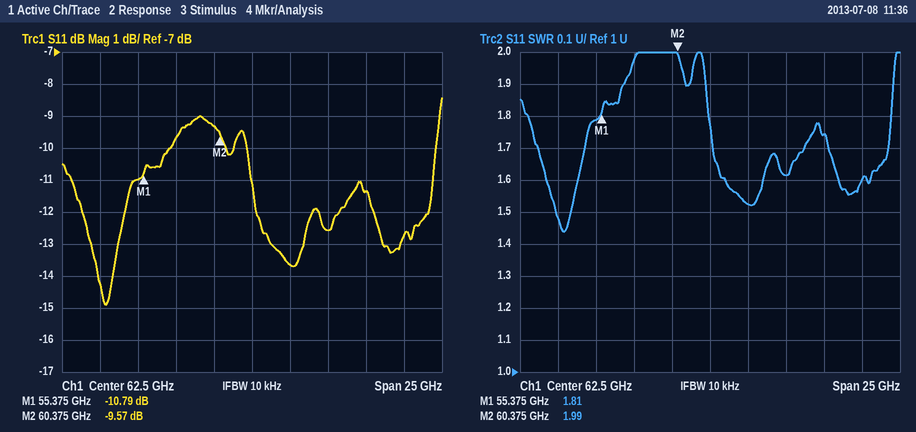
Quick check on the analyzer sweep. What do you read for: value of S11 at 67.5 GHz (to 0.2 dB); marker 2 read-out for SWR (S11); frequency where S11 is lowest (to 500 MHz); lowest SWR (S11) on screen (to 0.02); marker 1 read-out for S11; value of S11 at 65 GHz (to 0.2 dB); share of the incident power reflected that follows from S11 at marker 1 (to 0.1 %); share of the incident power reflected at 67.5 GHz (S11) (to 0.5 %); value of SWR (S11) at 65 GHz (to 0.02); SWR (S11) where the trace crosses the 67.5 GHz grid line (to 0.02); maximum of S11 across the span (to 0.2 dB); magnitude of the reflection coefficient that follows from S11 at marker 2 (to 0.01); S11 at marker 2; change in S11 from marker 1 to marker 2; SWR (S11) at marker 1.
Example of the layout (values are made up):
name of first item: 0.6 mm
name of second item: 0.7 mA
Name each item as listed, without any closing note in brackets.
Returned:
value of S11 at 67.5 GHz: -12.6 dB
marker 2 read-out for SWR: 1.99
frequency where S11 is lowest: 53.0 GHz
lowest SWR (S11) on screen: 1.44
marker 1 read-out for S11: -10.79 dB
value of S11 at 65 GHz: -13.6 dB
share of the incident power reflected that follows from S11 at marker 1: 8.3 %
share of the incident power reflected at 67.5 GHz (S11): 5.5 %
value of SWR (S11) at 65 GHz: 1.52
SWR (S11) where the trace crosses the 67.5 GHz grid line: 1.62
maximum of S11 across the span: -8.4 dB
magnitude of the reflection coefficient that follows from S11 at marker 2: 0.33
S11 at marker 2: -9.57 dB
change in S11 from marker 1 to marker 2: 1.22 dB
SWR (S11) at marker 1: 1.81
